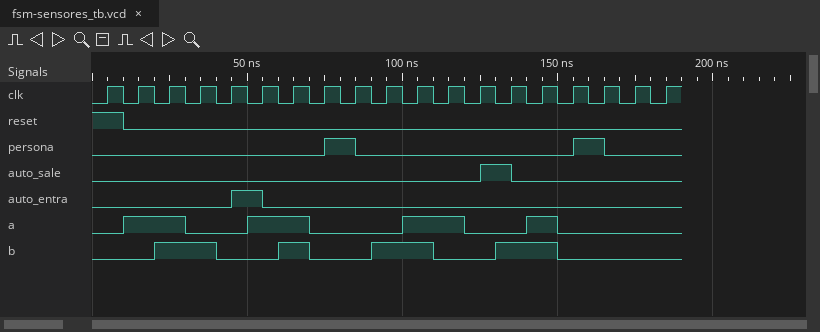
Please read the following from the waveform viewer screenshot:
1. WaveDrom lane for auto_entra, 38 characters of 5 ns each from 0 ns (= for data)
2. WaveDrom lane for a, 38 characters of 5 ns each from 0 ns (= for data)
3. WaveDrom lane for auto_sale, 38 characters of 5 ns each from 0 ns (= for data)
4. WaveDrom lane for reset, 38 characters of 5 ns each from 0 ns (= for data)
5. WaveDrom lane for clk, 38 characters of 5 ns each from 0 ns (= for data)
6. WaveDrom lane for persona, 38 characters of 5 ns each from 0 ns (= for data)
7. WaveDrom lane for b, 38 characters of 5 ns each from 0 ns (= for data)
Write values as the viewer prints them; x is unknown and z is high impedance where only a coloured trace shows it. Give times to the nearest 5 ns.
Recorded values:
{name: 'auto_entra', wave: '0........1.0..........................'}
{name: 'a', wave: '0.1...0...1...0.....1...0...1.0.......'}
{name: 'auto_sale', wave: '0........................1.0..........'}
{name: 'reset', wave: '1.0...................................'}
{name: 'clk', wave: '01010101010101010101010101010101010101'}
{name: 'persona', wave: '0..............1.0.............1.0....'}
{name: 'b', wave: '0...1...0...1.0...1...0...1...0.......'}
